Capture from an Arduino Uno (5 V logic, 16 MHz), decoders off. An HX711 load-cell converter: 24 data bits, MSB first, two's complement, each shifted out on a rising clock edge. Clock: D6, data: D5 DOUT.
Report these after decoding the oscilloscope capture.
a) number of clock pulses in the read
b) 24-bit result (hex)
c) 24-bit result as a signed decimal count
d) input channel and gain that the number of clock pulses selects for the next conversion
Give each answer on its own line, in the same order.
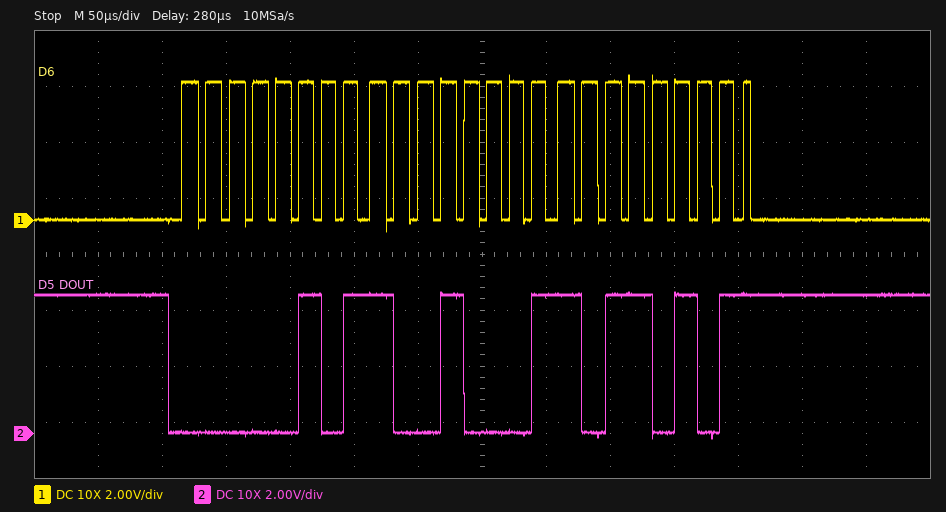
25
0x0591B5
364981
channel A, gain 128
